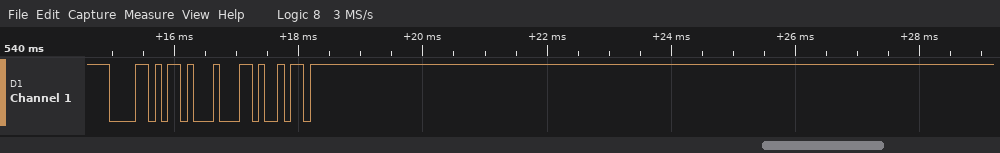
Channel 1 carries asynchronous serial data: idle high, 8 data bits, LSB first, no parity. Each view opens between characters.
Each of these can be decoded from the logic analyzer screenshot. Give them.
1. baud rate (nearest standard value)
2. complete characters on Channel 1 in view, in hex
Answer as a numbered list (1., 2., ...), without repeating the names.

1. 9600 baud
2. 58, 11, 69
